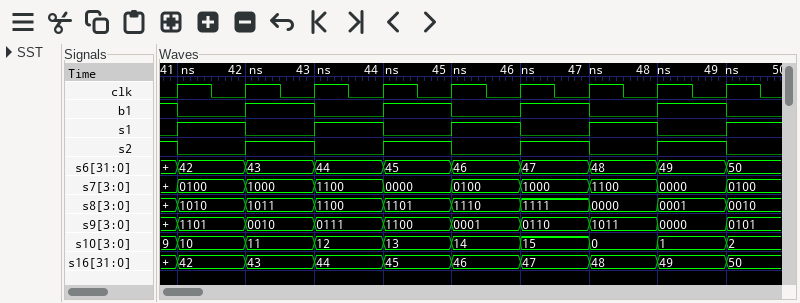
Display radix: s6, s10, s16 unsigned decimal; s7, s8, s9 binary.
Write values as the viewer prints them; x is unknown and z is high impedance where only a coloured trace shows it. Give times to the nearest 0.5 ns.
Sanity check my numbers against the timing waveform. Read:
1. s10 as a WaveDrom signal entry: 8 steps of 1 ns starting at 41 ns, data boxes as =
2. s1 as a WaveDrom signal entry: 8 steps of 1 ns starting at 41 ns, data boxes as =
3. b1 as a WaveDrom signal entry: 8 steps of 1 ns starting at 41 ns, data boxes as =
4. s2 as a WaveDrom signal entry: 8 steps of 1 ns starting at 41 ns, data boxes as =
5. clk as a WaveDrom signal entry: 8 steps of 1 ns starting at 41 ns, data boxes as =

{name: 's10', wave: '========', data: '10 11 12 13 14 15 0 1'}
{name: 's1', wave: '10101010'}
{name: 'b1', wave: '01010101'}
{name: 's2', wave: '01010101'}
{name: 'clk', wave: 'p.......'}
